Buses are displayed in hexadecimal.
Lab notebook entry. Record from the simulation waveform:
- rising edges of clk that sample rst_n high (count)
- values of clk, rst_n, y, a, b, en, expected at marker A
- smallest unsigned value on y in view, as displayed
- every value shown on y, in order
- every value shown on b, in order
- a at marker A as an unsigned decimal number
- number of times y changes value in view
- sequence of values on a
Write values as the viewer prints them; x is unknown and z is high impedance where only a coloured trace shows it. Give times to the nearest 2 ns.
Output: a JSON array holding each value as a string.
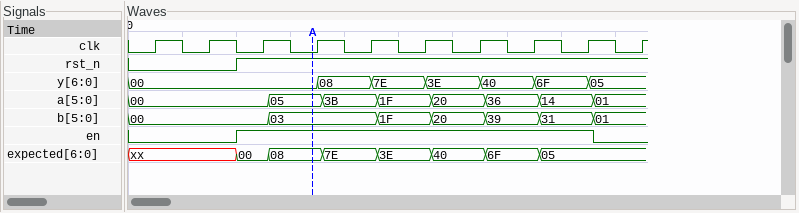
["8", "clk=0, rst_n=1, y=00, a=05, b=03, en=1, expected=08", "00", "00, 08, 7E, 3E, 40, 6F, 05", "00, 03, 1F, 20, 39, 31, 01", "5", "6", "00, 05, 3B, 1F, 20, 36, 14, 01"]
